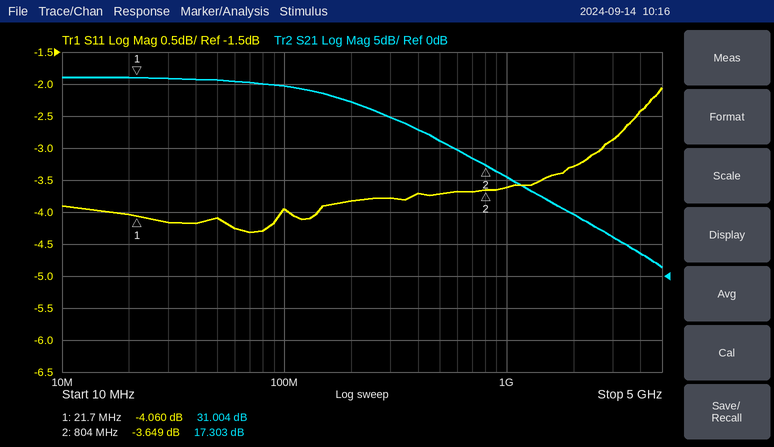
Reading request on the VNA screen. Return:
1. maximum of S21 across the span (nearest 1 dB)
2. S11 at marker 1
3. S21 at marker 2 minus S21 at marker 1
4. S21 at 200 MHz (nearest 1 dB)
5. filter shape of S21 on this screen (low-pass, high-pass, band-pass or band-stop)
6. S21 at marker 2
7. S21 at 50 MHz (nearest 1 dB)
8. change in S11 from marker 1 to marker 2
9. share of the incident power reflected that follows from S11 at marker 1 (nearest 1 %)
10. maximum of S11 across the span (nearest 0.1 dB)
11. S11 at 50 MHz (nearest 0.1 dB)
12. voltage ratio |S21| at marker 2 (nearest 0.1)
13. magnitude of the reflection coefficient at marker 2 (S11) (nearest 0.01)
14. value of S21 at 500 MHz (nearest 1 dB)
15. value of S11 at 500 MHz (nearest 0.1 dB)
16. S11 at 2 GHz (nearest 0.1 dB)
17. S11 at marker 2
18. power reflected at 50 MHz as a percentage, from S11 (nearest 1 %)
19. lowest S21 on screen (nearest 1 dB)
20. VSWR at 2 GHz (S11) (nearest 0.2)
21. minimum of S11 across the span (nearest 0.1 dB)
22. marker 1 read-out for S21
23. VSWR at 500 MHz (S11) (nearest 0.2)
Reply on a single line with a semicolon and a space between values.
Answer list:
31 dB; -4.060 dB; -13.701 dB; 27 dB; low-pass; 17.303 dB; 31 dB; 0.411 dB; 39 %; -2.1 dB; -4.1 dB; 7.3; 0.66; 21 dB; -3.7 dB; -3.3 dB; -3.649 dB; 39 %; 1 dB; 5.4; -4.3 dB; 31.004 dB; 4.8
